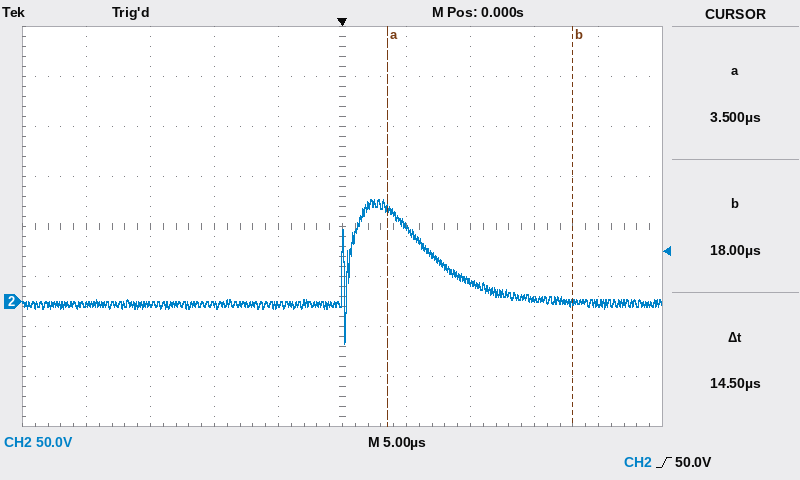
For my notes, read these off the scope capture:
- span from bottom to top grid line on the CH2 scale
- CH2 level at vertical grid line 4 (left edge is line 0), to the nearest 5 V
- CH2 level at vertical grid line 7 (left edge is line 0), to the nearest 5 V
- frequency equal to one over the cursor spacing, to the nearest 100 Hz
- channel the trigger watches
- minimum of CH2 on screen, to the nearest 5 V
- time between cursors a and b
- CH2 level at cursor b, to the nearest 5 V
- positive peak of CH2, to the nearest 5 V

400 V
-5 V
20 V
69.0 kHz
CH2
-40 V
14.5 µs
0 V
100 V
